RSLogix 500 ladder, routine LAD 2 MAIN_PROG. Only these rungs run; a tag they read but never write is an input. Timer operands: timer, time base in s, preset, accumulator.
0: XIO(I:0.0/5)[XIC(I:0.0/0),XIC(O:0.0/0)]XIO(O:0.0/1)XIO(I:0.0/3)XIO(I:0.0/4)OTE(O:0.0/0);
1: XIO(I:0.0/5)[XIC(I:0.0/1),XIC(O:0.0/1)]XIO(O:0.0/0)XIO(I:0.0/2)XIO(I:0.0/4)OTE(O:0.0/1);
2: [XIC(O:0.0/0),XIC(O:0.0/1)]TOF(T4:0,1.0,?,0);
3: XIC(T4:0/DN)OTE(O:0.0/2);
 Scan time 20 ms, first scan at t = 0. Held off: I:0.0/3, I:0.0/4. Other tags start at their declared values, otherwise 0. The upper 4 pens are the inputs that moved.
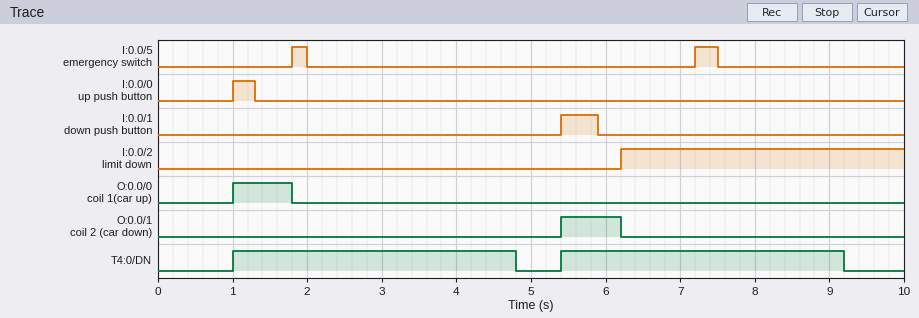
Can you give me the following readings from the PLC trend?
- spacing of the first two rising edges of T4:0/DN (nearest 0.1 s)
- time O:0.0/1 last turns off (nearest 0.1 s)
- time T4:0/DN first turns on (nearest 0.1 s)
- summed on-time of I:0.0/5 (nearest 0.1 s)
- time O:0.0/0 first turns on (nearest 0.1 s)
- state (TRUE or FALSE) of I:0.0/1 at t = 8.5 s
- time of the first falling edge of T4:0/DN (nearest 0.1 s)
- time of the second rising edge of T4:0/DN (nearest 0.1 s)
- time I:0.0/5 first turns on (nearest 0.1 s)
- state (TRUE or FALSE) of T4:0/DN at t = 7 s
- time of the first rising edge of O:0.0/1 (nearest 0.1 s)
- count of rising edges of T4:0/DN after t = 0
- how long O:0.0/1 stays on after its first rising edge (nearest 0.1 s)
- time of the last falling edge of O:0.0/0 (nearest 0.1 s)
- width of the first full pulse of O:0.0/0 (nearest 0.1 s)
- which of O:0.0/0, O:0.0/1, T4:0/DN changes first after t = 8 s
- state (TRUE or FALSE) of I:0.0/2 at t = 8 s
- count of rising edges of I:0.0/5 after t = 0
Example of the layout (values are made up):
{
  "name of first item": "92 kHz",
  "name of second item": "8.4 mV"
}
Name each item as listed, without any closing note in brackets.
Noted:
{
  "spacing of the first two rising edges of T4:0/DN": "4.4 s",
  "time O:0.0/1 last turns off": "6.2 s",
  "time T4:0/DN first turns on": "1.0 s",
  "summed on-time of I:0.0/5": "0.5 s",
  "time O:0.0/0 first turns on": "1.0 s",
  "state (TRUE or FALSE) of I:0.0/1 at t = 8.5 s": "FALSE",
  "time of the first falling edge of T4:0/DN": "4.8 s",
  "time of the second rising edge of T4:0/DN": "5.4 s",
  "time I:0.0/5 first turns on": "1.8 s",
  "state (TRUE or FALSE) of T4:0/DN at t = 7 s": "TRUE",
  "time of the first rising edge of O:0.0/1": "5.4 s",
  "count of rising edges of T4:0/DN after t = 0": "2",
  "how long O:0.0/1 stays on after its first rising edge": "0.8 s",
  "time of the last falling edge of O:0.0/0": "1.8 s",
  "width of the first full pulse of O:0.0/0": "0.8 s",
  "which of O:0.0/0, O:0.0/1, T4:0/DN changes first after t = 8 s": "T4:0/DN",
  "state (TRUE or FALSE) of I:0.0/2 at t = 8 s": "TRUE",
  "count of rising edges of I:0.0/5 after t = 0": "2"
}
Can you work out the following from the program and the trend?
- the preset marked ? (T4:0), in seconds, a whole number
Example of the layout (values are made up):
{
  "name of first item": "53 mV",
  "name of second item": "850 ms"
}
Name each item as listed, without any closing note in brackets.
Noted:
{
  "the preset marked ? (T4:0), in seconds, a whole number": "3 s"
}
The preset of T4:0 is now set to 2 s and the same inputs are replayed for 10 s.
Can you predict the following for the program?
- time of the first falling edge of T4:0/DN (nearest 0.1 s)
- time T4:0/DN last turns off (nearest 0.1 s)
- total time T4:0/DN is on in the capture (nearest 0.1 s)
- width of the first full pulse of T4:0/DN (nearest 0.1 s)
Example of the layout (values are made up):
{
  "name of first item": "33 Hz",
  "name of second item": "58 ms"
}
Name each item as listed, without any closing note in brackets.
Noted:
{
  "time of the first falling edge of T4:0/DN": "3.8 s",
  "time T4:0/DN last turns off": "8.2 s",
  "total time T4:0/DN is on in the capture": "5.6 s",
  "width of the first full pulse of T4:0/DN": "2.8 s"
}
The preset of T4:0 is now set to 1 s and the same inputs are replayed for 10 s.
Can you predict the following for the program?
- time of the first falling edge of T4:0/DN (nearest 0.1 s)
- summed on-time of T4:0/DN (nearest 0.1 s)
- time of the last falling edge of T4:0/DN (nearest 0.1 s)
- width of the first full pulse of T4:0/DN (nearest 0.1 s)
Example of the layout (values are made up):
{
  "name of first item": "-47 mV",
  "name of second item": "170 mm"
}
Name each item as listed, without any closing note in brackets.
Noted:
{
  "time of the first falling edge of T4:0/DN": "2.8 s",
  "summed on-time of T4:0/DN": "3.6 s",
  "time of the last falling edge of T4:0/DN": "7.2 s",
  "width of the first full pulse of T4:0/DN": "1.8 s"
}
